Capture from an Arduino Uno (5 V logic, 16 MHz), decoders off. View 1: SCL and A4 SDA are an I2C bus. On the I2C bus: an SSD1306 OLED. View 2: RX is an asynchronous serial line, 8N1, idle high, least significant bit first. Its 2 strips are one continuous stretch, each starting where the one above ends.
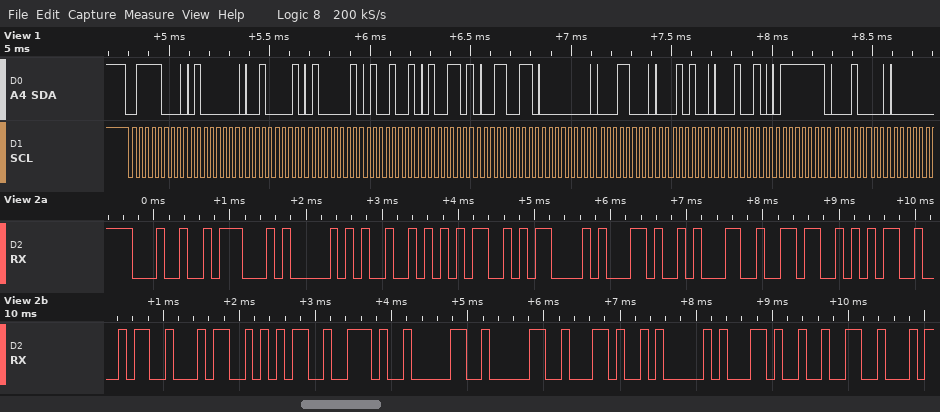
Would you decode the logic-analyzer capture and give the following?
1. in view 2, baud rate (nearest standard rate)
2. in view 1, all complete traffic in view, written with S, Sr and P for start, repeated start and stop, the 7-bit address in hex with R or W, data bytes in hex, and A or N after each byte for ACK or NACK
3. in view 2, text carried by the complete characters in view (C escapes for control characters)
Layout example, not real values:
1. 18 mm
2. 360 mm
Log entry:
1. 9600 baud
2. S 3CW A 40 A 21 A 41 A 49 A 4D A 33 A 00 A 18 A 14 A 12 A 7F A 10 A
3. "$GPRMC,165445.00,A,2"
